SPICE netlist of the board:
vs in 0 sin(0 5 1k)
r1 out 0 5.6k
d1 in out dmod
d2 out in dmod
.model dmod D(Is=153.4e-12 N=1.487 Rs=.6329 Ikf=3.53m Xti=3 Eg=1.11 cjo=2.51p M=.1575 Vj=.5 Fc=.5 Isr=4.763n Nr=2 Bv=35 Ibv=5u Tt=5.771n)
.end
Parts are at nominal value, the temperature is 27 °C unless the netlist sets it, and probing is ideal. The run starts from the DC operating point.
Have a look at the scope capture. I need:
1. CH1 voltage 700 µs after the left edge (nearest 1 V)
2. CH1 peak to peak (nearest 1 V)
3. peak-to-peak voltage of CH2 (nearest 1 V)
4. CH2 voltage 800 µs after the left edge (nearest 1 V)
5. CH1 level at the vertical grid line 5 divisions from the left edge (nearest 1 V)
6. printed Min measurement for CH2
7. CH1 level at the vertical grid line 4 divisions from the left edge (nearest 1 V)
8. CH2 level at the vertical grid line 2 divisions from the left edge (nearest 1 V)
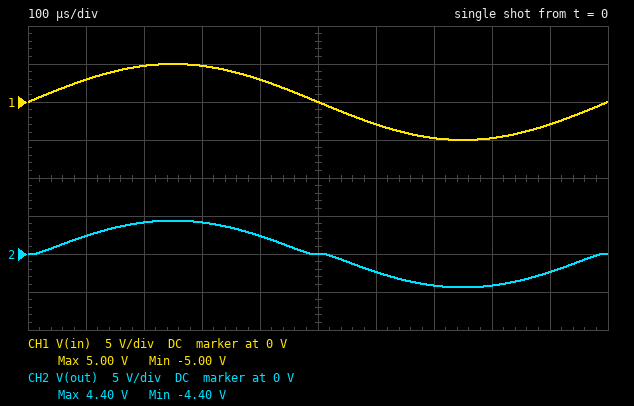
-5 V
10 V
9 V
-4 V
0 V
-4.40 V
3 V
4 V
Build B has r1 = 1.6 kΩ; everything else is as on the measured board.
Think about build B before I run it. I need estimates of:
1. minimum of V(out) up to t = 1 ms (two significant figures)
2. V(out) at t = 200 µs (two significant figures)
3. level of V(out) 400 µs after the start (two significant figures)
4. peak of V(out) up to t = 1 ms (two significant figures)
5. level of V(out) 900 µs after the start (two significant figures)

-4.3 V
4.1 V
2.3 V
4.3 V
-2.3 V
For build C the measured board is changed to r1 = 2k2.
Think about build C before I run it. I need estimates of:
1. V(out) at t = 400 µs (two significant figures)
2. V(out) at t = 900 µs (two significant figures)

2.3 V
-2.3 V
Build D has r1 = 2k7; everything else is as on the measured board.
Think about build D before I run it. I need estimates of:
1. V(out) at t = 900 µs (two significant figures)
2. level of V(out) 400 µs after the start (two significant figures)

-2.3 V
2.3 V
